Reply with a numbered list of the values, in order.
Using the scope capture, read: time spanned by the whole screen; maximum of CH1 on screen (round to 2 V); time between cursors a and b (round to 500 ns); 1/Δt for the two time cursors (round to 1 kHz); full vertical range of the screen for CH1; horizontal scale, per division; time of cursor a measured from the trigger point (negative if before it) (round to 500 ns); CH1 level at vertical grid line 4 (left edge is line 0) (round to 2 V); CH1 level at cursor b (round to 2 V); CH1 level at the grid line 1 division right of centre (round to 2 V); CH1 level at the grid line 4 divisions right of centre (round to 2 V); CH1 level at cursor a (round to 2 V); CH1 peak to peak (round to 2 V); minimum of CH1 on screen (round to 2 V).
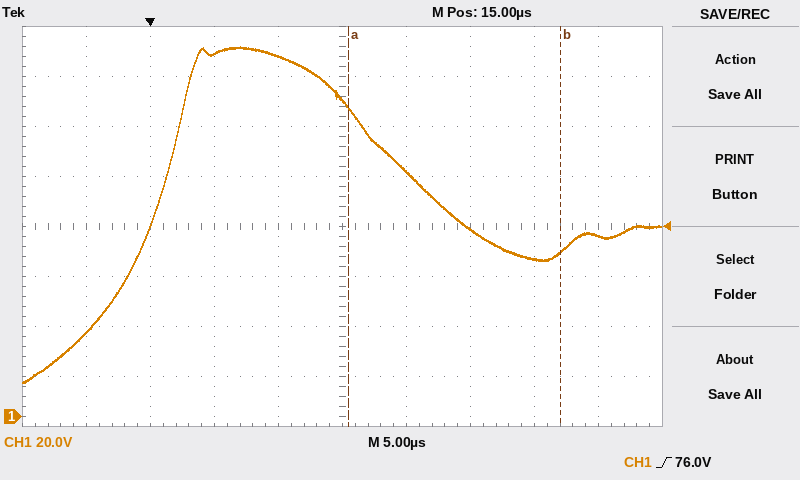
1. 50 µs
2. 148 V
3. 16.5 µs
4. 61 kHz
5. 160 V
6. 5 µs
7. +15.5 µs
8. 144 V
9. 66 V
10. 98 V
11. 72 V
12. 124 V
13. 134 V
14. 14 V
